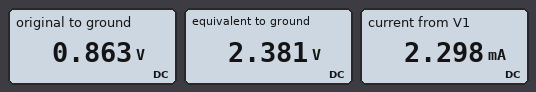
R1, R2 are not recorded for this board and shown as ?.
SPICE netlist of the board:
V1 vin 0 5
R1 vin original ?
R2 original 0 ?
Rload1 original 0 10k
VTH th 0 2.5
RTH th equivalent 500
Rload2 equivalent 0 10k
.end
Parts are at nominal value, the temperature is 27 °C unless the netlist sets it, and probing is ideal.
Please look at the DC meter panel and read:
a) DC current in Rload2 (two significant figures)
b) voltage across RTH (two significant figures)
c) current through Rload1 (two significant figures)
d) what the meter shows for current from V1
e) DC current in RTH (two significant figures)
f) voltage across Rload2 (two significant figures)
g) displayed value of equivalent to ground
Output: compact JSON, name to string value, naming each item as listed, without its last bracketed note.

{"DC current in Rload2": "240 µA", "voltage across RTH": "120 mV", "current through Rload1": "86 µA", "what the meter shows for current from V1": "2.298 mA", "DC current in RTH": "240 µA", "voltage across Rload2": "2.4 V", "displayed value of equivalent to ground": "2.381 V"}
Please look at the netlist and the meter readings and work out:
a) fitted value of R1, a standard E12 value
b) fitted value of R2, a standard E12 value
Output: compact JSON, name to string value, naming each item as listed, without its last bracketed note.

{"fitted value of R1, a standard E12 value": "1.8 kΩ", "fitted value of R2, a standard E12 value": "390 Ω"}
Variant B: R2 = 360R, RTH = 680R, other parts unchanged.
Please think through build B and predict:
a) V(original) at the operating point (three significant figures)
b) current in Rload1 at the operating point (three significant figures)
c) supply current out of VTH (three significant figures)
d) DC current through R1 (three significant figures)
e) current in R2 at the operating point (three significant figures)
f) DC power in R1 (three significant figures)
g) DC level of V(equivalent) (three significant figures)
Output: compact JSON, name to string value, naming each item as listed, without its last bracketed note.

{"V(original) at the operating point": "809 mV", "current in Rload1 at the operating point": "80.9 µA", "supply current out of VTH": "234 µA", "DC current through R1": "2.33 mA", "current in R2 at the operating point": "2.25 mA", "DC power in R1": "9.76 mW", "DC level of V(equivalent)": "2.34 V"}
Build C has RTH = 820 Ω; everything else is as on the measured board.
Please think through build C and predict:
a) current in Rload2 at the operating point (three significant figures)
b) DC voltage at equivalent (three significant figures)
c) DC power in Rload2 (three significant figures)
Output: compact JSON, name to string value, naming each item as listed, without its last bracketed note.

{"current in Rload2 at the operating point": "231 µA", "DC voltage at equivalent": "2.31 V", "DC power in Rload2": "534 µW"}
